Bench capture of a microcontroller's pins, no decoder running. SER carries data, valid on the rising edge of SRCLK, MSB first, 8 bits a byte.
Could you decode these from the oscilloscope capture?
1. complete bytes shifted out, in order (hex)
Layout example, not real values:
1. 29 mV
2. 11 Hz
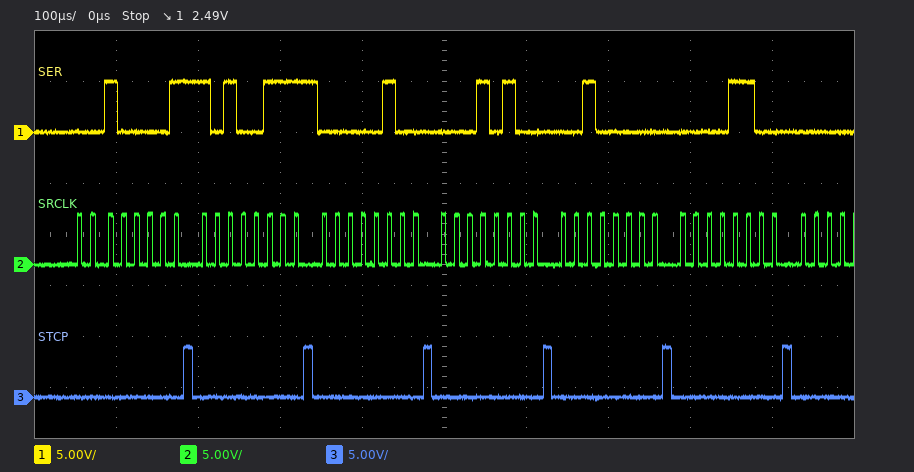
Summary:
1. 21 A7 04 14 20 0C
